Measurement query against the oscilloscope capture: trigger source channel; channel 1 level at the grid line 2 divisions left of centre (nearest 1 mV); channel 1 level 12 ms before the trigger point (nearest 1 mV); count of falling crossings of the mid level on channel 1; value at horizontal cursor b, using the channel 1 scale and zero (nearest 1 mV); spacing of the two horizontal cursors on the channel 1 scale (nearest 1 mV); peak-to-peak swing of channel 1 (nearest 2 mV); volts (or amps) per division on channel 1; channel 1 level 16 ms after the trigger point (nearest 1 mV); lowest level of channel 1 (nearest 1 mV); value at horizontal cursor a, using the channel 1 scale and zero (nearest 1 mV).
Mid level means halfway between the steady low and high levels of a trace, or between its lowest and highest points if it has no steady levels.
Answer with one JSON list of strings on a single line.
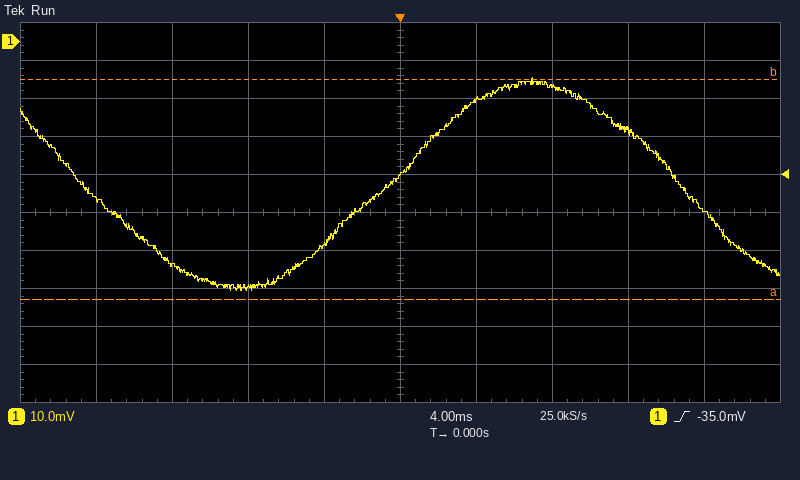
["channel 1", "-65 mV", "-58 mV", "2", "-10 mV", "58 mV", "56 mV", "10 mV", "-45 mV", "-66 mV", "-68 mV"]
